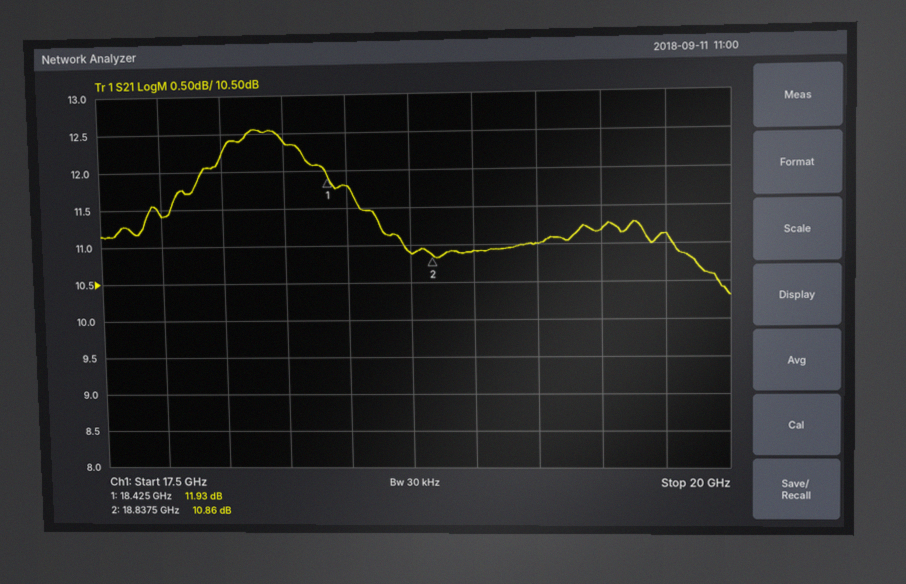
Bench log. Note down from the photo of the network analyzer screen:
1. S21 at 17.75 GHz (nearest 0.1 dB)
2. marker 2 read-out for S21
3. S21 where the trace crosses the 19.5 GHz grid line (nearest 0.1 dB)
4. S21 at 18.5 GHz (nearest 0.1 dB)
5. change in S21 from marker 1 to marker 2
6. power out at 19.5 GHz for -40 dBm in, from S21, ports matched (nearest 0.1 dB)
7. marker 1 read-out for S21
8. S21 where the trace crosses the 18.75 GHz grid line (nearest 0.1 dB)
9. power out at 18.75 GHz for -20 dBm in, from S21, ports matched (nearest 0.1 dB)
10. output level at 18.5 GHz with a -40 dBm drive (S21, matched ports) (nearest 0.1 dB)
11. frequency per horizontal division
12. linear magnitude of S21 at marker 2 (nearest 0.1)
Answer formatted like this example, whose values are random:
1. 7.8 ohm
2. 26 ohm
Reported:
1. 11.4 dB
2. 10.86 dB
3. 11.2 dB
4. 11.8 dB
5. -1.07 dB
6. -28.8 dBm
7. 11.93 dB
8. 10.9 dB
9. -9.1 dBm
10. -28.2 dBm
11. 250 MHz
12. 3.5
